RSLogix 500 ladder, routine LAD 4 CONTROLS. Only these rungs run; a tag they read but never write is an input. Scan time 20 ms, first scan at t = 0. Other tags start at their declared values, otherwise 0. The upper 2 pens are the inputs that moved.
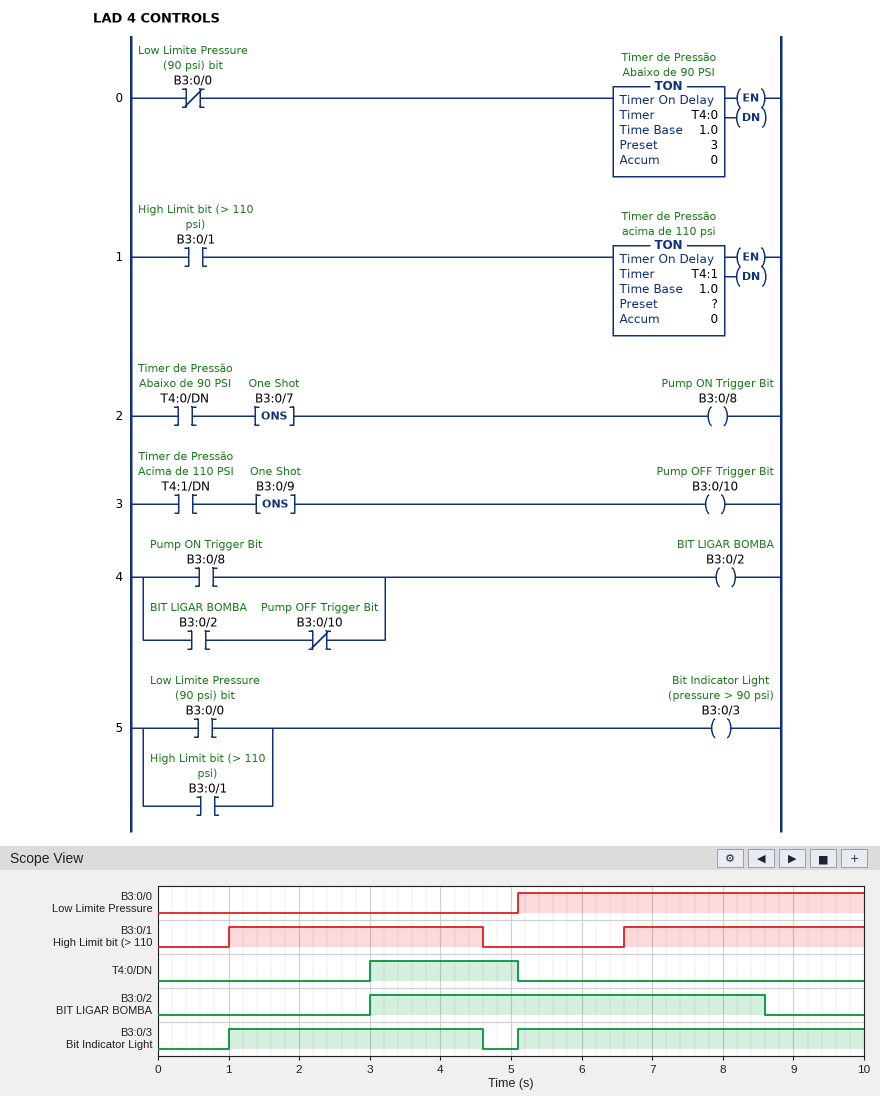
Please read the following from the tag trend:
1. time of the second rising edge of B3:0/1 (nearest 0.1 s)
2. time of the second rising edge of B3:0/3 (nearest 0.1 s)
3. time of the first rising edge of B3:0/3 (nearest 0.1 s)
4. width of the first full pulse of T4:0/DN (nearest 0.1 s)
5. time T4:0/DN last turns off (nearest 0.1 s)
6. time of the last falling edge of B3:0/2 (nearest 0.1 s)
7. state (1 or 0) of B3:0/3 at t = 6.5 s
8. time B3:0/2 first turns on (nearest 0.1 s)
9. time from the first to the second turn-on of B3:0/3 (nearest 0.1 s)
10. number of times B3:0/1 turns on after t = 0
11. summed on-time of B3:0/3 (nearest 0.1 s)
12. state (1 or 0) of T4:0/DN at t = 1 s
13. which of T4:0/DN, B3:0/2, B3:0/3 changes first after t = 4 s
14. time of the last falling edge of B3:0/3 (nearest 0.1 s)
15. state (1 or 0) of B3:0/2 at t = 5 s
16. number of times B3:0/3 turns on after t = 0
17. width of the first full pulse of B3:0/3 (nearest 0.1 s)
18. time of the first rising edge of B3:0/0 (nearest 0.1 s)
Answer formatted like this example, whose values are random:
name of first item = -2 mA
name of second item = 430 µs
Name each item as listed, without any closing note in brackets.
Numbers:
time of the second rising edge of B3:0/1 = 6.6 s
time of the second rising edge of B3:0/3 = 5.1 s
time of the first rising edge of B3:0/3 = 1.0 s
width of the first full pulse of T4:0/DN = 2.1 s
time T4:0/DN last turns off = 5.1 s
time of the last falling edge of B3:0/2 = 8.6 s
state (1 or 0) of B3:0/3 at t = 6.5 s = 1
time B3:0/2 first turns on = 3.0 s
time from the first to the second turn-on of B3:0/3 = 4.1 s
number of times B3:0/1 turns on after t = 0 = 2
summed on-time of B3:0/3 = 8.5 s
state (1 or 0) of T4:0/DN at t = 1 s = 0
which of T4:0/DN, B3:0/2, B3:0/3 changes first after t = 4 s = B3:0/3
time of the last falling edge of B3:0/3 = 4.6 s
state (1 or 0) of B3:0/2 at t = 5 s = 1
number of times B3:0/3 turns on after t = 0 = 2
width of the first full pulse of B3:0/3 = 3.6 s
time of the first rising edge of B3:0/0 = 5.1 s
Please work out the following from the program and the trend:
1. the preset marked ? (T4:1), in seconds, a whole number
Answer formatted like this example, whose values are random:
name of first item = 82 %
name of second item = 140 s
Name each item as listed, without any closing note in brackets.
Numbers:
the preset marked ? (T4:1), in seconds, a whole number = 2 s
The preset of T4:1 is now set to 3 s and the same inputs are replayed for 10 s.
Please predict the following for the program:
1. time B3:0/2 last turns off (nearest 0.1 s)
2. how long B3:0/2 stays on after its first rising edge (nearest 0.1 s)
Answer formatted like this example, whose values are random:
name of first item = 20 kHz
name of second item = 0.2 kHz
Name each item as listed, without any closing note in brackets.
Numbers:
time B3:0/2 last turns off = 4.0 s
how long B3:0/2 stays on after its first rising edge = 1.0 s
